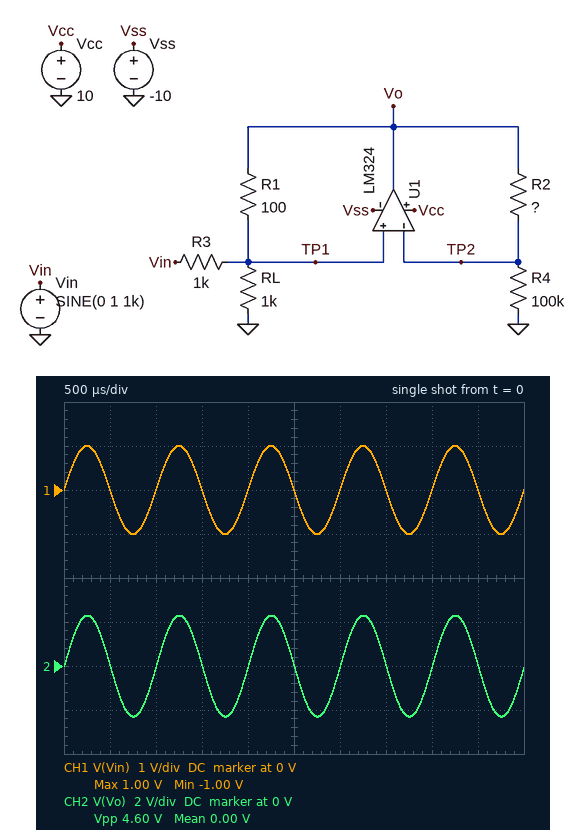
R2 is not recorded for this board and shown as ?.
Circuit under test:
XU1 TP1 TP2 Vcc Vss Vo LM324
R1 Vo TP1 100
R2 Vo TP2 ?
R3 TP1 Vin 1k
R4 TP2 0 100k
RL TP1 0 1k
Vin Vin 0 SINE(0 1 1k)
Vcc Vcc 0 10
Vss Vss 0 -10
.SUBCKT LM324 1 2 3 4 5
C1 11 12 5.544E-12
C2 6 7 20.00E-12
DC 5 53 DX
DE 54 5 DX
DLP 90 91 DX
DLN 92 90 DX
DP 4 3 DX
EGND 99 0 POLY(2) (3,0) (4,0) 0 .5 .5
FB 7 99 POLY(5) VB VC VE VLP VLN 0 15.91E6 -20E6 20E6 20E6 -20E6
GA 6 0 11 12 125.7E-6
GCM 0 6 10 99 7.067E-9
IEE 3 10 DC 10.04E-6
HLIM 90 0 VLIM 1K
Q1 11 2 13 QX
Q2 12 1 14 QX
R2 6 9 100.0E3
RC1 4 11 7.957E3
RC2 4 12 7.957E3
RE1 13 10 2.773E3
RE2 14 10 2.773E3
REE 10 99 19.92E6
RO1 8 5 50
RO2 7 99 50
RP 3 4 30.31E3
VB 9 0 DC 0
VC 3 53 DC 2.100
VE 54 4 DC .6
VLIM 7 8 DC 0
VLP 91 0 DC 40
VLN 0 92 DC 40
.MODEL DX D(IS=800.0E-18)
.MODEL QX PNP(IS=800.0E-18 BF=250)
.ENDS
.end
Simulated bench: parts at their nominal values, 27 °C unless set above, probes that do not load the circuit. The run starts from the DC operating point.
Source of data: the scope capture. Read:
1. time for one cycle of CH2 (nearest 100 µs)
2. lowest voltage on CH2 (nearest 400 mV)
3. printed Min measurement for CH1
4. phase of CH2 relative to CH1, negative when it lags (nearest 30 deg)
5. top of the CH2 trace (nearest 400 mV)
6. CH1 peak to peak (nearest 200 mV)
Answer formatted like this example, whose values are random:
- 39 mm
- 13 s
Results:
- 1.0 ms
- -2.4 V
- -1.00 V
- 0 deg
- 2.4 V
- 2.0 V
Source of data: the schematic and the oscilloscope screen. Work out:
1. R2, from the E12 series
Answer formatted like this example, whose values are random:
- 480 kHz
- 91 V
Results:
- 15 kΩ
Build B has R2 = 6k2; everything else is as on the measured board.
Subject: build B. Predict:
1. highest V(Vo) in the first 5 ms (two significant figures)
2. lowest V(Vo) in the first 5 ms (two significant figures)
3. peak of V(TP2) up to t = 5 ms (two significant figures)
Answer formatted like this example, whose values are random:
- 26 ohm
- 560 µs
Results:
- 770 mV
- -770 mV
- 720 mV
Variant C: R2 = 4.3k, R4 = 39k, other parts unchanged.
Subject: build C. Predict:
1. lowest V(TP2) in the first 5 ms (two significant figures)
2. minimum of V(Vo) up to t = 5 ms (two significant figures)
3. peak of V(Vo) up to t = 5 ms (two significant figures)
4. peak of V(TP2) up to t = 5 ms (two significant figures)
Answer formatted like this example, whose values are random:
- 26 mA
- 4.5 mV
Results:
- -1.1 V
- -1.2 V
- 1.2 V
- 1.1 V
